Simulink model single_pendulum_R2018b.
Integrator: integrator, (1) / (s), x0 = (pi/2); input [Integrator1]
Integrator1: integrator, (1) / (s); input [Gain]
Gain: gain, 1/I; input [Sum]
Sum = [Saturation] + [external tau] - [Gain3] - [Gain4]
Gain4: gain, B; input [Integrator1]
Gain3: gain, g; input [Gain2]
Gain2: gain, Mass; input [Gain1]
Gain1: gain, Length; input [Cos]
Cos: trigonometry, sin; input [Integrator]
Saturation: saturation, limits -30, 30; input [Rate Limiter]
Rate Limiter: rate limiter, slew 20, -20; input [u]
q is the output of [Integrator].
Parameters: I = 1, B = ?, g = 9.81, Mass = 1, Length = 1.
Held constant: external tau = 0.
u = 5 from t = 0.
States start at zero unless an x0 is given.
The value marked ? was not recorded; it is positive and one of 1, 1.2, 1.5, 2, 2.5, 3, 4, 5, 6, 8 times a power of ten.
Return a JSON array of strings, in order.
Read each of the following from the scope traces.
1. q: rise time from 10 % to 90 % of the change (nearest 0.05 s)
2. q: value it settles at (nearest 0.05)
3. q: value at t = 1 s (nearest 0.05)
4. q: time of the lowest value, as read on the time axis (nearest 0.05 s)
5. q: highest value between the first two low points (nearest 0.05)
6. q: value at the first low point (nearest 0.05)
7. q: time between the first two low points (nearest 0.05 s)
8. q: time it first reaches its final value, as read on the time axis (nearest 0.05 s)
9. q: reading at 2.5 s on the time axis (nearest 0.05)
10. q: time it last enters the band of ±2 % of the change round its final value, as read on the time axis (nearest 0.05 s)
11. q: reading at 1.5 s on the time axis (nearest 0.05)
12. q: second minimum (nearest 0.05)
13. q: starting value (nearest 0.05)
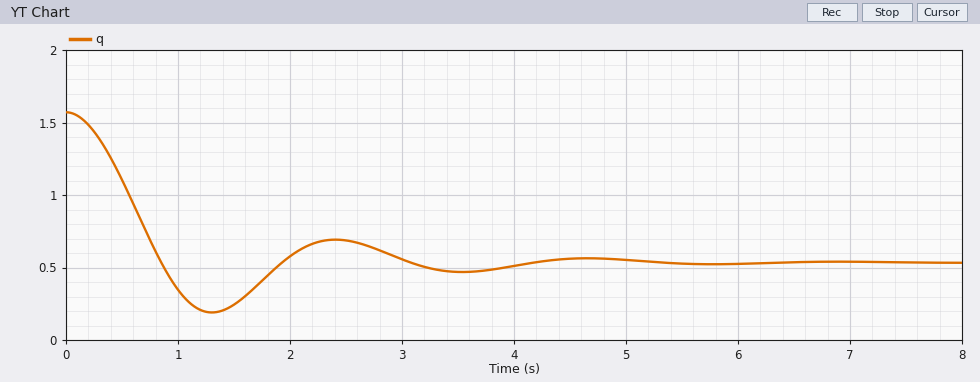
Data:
["0.55 s", "0.55", "0.35", "1.30 s", "0.70", "0.20", "2.25 s", "0.85 s", "0.70", "4.95 s", "0.25", "0.45", "1.55"]
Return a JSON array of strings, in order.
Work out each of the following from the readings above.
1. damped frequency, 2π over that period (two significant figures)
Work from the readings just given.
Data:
["2.8 rad/s"]
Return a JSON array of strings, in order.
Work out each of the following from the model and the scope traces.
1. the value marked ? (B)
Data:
["1.5"]
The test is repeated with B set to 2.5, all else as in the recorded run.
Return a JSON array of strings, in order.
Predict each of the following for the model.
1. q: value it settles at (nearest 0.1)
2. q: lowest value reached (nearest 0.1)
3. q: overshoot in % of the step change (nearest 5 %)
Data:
["0.5", "0.4", "15 %"]
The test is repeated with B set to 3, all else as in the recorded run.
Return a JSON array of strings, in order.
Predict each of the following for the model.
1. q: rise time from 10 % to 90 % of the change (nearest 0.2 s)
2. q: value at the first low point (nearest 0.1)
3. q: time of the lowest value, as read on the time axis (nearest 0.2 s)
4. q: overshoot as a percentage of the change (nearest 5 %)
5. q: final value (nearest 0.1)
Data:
["0.8 s", "0.4", "1.6 s", "10 %", "0.5"]
